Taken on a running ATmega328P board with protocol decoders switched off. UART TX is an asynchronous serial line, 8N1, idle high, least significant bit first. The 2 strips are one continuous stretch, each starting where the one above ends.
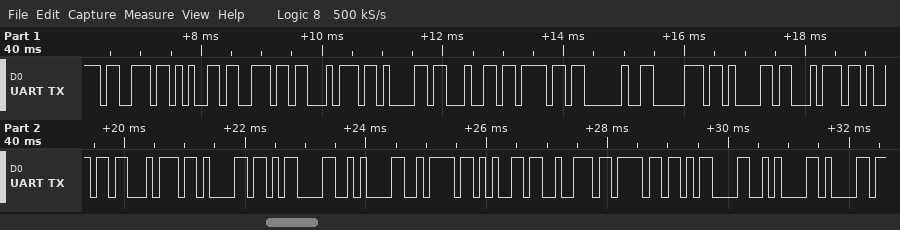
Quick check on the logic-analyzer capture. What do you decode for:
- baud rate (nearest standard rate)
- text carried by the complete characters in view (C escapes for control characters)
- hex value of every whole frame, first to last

9600 baud
"sentado patita\r\nzero\r\na"
0x73 0x65 0x6E 0x74 0x61 0x64 0x6F 0x20 0x70 0x61 0x74 0x69 0x74 0x61 0x0D 0x0A 0x7A 0x65 0x72 0x6F 0x0D 0x0A 0x61
